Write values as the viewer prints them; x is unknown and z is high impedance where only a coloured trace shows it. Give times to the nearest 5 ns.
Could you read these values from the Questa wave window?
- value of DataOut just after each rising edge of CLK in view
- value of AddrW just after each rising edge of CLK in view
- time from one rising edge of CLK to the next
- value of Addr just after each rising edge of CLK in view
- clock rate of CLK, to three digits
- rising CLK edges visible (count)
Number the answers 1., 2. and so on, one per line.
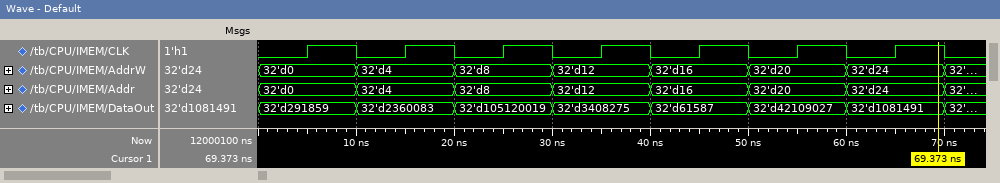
1. 32'd291859, 32'd2360083, 32'd105120019, 32'd3408275, 32'd61587, 32'd42109027, 32'd1081491
2. 32'd0, 32'd4, 32'd8, 32'd12, 32'd16, 32'd20, 32'd24
3. 10 ns
4. 32'd0, 32'd4, 32'd8, 32'd12, 32'd16, 32'd20, 32'd24
5. 100 MHz
6. 7
